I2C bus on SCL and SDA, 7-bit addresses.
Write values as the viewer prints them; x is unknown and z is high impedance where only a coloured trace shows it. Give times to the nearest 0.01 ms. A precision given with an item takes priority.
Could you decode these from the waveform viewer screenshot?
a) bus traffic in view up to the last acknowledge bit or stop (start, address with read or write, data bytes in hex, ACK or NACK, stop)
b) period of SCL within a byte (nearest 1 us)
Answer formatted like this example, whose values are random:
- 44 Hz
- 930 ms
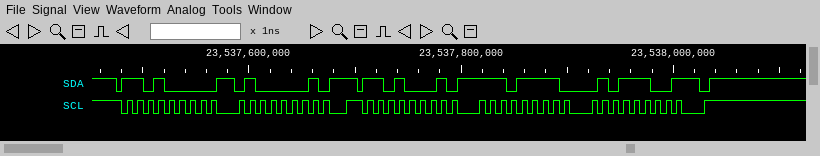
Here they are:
- start, address 68 write ACK, 41 ACK, repeated start, address 68 read ACK, EF ACK, 5C NACK, stop
- 10 us
